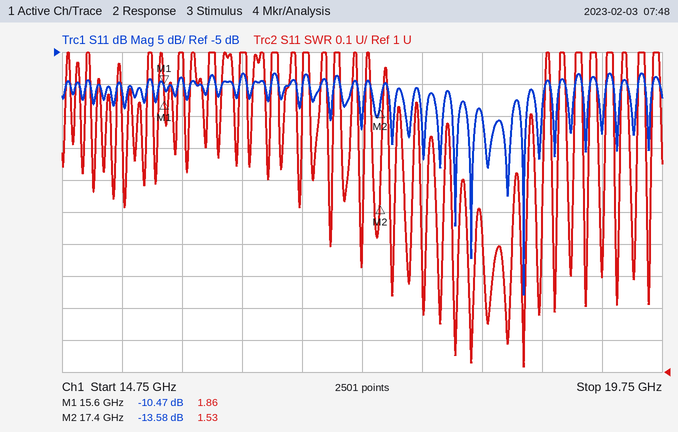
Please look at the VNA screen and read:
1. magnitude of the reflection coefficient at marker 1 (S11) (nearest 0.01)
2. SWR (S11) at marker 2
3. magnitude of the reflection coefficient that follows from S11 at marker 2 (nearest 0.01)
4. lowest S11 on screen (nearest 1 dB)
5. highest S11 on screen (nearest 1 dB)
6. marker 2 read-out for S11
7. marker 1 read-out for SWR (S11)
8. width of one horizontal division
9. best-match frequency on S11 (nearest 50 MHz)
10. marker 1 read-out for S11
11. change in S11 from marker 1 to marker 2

0.30
1.53
0.21
-43 dB
-8 dB
-13.58 dB
1.86
500 MHz
18.60 GHz
-10.47 dB
-3.11 dB
